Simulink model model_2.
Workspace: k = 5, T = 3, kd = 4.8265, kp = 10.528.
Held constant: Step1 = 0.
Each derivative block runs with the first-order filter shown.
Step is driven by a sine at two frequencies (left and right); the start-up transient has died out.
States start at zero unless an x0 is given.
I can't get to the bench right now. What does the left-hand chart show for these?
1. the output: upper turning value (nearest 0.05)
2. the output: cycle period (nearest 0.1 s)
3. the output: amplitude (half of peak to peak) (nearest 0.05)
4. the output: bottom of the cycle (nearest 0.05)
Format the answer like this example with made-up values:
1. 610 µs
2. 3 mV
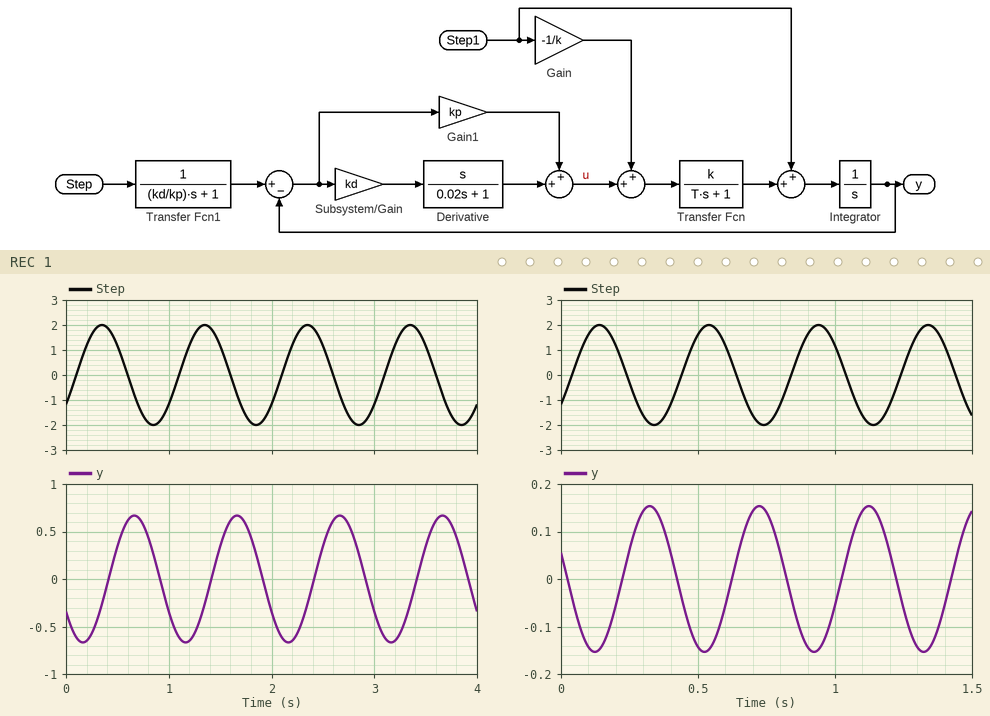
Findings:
1. 0.65
2. 1.0 s
3. 0.65
4. -0.65
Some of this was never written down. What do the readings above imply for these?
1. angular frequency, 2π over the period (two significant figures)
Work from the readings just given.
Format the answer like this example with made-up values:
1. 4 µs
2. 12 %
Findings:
1. 6.3 rad/s
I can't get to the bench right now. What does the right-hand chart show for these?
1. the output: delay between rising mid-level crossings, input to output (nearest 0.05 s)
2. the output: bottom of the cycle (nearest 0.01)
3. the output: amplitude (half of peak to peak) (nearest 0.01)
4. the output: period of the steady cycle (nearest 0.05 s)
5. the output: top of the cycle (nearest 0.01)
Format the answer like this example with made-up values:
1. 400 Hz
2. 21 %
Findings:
1. 0.20 s
2. -0.15
3. 0.15
4. 0.40 s
5. 0.15
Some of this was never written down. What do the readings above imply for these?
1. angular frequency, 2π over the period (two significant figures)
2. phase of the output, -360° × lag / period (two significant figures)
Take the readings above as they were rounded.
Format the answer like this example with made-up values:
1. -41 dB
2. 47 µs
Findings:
1. 16 rad/s
2. -180°
